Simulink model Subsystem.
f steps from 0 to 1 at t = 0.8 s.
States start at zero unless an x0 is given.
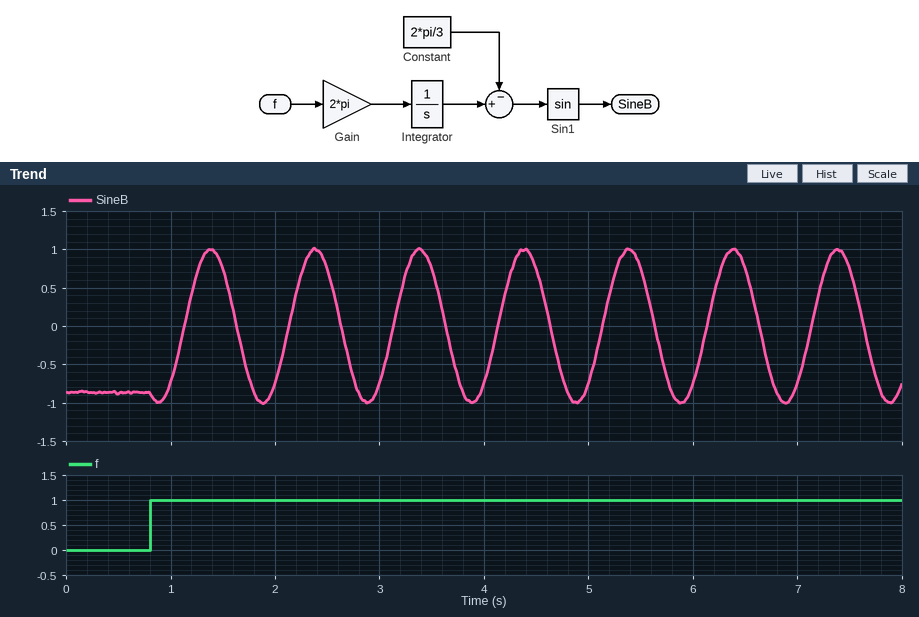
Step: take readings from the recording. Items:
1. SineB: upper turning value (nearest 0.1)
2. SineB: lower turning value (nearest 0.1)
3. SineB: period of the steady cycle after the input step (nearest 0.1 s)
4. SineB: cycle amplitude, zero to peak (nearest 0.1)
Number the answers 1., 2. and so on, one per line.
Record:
1. 1.0
2. -1.0
3. 1.0 s
4. 1.0
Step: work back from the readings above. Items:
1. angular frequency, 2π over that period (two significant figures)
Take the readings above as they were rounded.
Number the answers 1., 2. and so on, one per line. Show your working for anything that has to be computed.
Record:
1. 2π / 1 = 6.3 rad/s
